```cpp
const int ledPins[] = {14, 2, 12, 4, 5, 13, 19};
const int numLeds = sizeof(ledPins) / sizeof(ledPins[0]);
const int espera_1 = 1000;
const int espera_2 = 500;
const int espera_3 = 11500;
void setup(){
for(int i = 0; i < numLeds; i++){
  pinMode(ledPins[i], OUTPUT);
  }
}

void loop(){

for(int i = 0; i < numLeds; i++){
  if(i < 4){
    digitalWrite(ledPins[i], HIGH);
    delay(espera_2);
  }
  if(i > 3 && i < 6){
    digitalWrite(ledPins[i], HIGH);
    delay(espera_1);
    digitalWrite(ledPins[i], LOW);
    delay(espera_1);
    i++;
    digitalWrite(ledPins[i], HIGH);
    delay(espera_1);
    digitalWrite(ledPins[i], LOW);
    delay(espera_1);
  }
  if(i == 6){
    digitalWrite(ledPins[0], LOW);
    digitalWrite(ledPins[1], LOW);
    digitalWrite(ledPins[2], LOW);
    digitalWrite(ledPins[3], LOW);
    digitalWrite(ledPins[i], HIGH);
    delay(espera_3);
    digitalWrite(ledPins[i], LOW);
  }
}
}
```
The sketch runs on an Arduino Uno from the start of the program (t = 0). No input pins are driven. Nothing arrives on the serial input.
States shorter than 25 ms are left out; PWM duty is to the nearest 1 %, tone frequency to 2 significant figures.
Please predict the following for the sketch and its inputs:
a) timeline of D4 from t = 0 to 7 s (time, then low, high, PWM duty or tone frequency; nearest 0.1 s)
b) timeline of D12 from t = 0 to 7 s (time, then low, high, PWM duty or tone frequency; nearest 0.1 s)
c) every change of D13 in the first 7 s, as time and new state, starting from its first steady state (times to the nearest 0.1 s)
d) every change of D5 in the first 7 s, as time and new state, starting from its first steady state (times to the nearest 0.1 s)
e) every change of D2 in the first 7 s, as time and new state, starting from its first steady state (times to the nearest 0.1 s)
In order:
0 s low; 1.5 s high; 6 s low
0 s low; 1 s high; 6 s low
0 s low; 4 s high; 5 s low
0 s low; 2 s high; 3 s low
0 s low; 0.5 s high; 6 s low
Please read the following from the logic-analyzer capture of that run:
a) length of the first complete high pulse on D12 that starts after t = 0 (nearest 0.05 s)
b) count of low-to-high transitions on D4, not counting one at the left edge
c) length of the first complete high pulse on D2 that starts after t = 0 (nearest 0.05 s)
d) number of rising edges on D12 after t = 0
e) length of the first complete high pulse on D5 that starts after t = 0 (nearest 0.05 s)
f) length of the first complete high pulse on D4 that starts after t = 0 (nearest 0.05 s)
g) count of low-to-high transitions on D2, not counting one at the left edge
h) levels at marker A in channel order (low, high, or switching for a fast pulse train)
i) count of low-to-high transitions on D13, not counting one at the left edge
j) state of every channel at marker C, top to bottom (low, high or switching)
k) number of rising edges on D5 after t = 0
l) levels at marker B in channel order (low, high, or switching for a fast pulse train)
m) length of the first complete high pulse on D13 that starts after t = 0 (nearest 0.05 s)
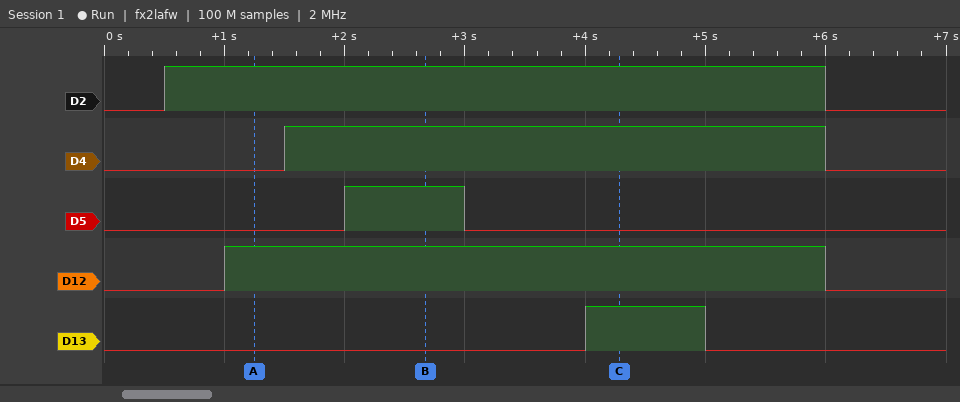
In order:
5.00 s
1
5.50 s
1
1.00 s
4.50 s
1
D2 high, D4 low, D5 low, D12 high, D13 low
1
D2 high, D4 high, D5 low, D12 high, D13 high
1
D2 high, D4 high, D5 high, D12 high, D13 low
1.00 s
